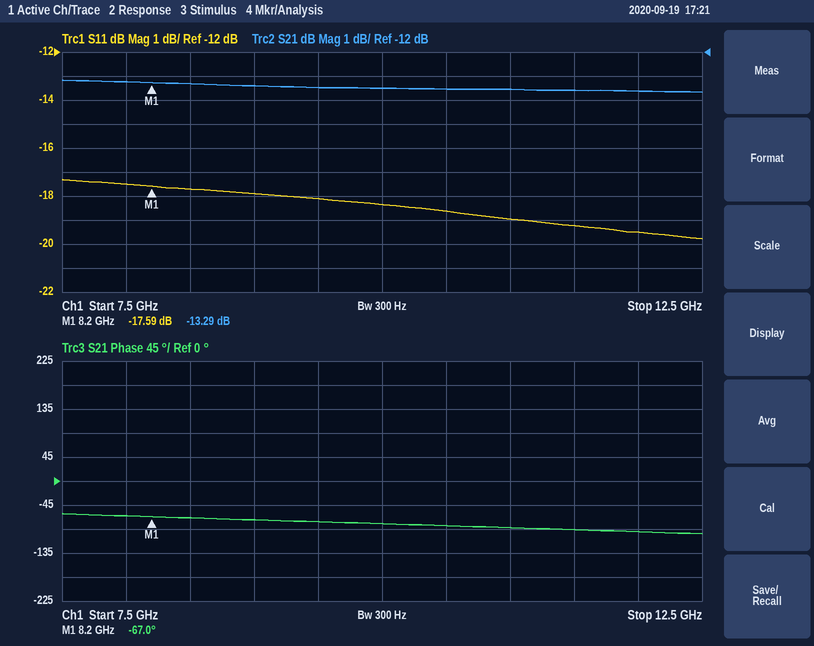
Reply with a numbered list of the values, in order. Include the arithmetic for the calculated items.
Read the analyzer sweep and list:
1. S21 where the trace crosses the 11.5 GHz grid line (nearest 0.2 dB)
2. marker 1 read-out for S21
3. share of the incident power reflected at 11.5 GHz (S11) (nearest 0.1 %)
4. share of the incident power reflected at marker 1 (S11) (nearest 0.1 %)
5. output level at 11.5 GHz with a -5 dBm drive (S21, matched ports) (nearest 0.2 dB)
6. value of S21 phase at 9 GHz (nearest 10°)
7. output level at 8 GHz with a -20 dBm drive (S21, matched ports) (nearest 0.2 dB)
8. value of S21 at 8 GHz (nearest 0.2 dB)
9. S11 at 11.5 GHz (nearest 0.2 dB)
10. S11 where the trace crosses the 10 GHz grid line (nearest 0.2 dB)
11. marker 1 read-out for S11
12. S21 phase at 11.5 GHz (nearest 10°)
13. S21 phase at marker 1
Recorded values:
1. -13.6 dB
2. -13.29 dB
3. 10^(-19.2/10) ≈ 1.2 %
4. 10^(-17.59/10) ≈ 1.7 %
5. -5 dBm + (-13.6 dB) = -18.6 dBm
6. -70°
7. -20 dBm + (-13.2 dB) = -33.2 dBm
8. -13.2 dB
9. -19.2 dB
10. -18.4 dB
11. -17.59 dB
12. -90°
13. -67.0°
